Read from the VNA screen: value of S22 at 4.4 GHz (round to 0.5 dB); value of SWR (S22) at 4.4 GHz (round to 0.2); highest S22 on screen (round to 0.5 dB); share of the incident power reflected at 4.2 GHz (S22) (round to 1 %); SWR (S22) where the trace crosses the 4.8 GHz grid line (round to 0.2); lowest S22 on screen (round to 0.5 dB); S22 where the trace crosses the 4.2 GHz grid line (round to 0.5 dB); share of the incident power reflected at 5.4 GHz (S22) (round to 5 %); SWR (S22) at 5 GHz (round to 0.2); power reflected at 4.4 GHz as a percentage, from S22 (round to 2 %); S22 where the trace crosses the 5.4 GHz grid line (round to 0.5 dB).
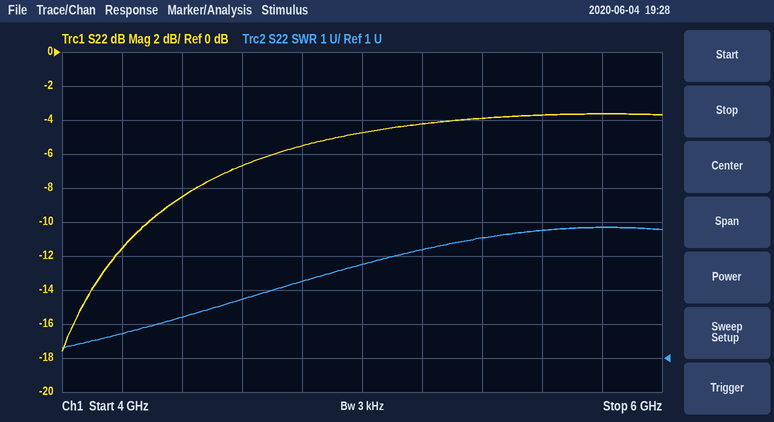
-8.5 dB
2.2
-3.5 dB
7 %
3.2
-17.5 dB
-11.5 dB
40 %
3.8
14 %
-4.0 dB
